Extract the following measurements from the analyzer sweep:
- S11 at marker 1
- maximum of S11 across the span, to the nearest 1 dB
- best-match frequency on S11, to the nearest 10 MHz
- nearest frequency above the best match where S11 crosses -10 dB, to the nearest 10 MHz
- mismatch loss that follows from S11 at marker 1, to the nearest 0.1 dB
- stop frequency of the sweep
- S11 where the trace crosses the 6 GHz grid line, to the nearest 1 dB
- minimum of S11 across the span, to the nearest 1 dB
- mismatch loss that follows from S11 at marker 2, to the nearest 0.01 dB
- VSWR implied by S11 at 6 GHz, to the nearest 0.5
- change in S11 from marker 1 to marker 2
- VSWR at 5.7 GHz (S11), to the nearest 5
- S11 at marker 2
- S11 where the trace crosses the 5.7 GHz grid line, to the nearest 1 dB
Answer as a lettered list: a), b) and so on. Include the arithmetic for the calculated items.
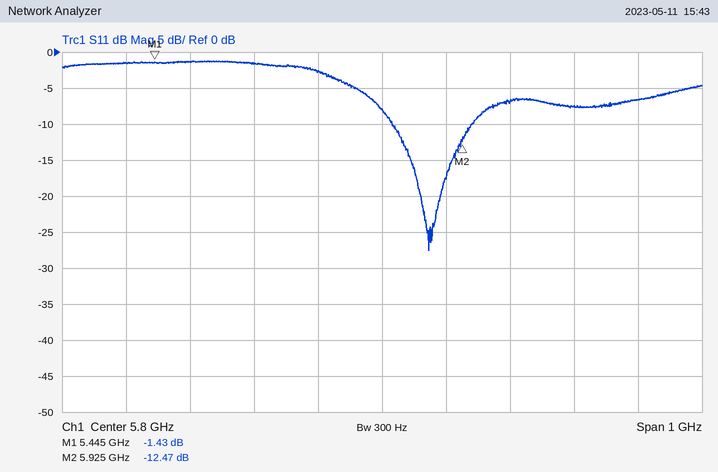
a) -1.43 dB
b) -1 dB
c) 5.87 GHz
d) 5.94 GHz
e) −10 log10(1 − 10^(-1.43/10)) ≈ 5.5 dB
f) 6.3 GHz
g) -7 dB
h) -28 dB
i) −10 log10(1 − 10^(-12.47/10)) ≈ 0.25 dB
j) |Γ| = 10^(-7/20) = 0.4467; VSWR = (1 + 0.4467)/(1 − 0.4467) ≈ 2.61, so 2.5 to the nearest 0.5
k) -12.47 − (-1.43) = -11.04 dB
l) |Γ| = 10^(-3/20) = 0.7079; VSWR = (1 + 0.7079)/(1 − 0.7079) ≈ 5.85, so 5 to the nearest 5
m) -12.47 dB
n) -3 dB
